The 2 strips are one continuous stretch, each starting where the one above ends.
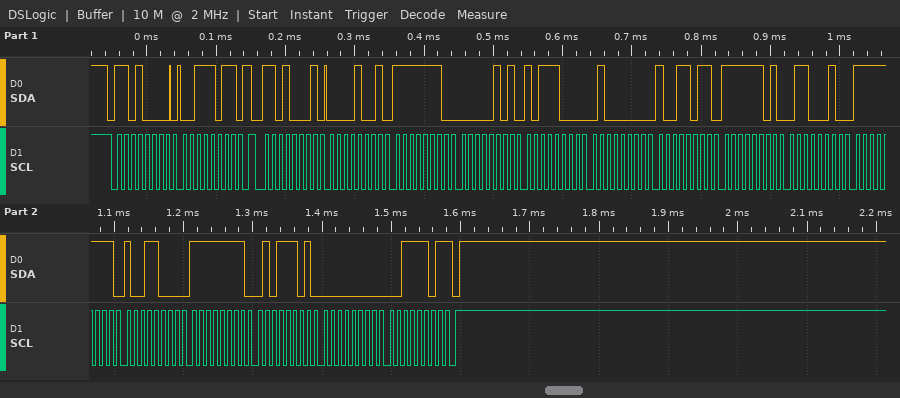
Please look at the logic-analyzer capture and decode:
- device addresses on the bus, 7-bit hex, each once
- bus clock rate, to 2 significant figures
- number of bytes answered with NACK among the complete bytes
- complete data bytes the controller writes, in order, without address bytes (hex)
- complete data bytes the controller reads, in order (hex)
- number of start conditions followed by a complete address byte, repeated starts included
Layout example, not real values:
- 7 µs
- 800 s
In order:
- 0x68
- 100 kHz
- 1
- 3B
- 09 FE 05 B8 40 9B FD 62 FF 98 FF 5D 00 3D
- 2
